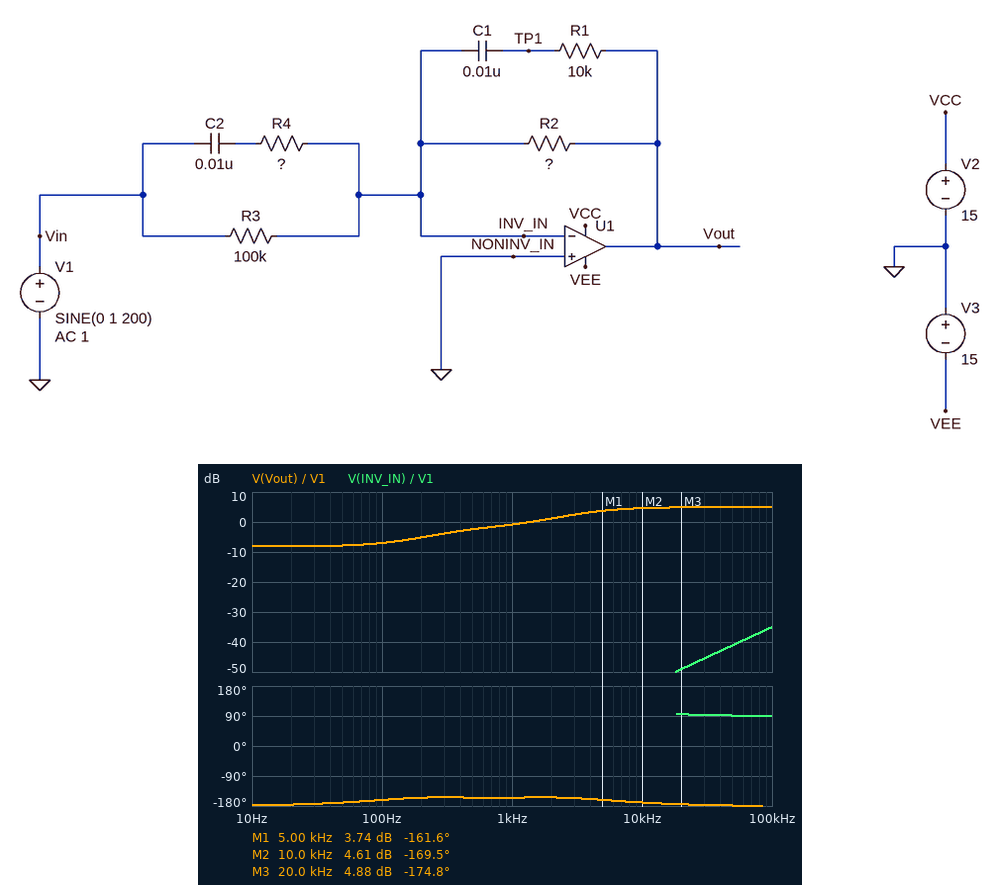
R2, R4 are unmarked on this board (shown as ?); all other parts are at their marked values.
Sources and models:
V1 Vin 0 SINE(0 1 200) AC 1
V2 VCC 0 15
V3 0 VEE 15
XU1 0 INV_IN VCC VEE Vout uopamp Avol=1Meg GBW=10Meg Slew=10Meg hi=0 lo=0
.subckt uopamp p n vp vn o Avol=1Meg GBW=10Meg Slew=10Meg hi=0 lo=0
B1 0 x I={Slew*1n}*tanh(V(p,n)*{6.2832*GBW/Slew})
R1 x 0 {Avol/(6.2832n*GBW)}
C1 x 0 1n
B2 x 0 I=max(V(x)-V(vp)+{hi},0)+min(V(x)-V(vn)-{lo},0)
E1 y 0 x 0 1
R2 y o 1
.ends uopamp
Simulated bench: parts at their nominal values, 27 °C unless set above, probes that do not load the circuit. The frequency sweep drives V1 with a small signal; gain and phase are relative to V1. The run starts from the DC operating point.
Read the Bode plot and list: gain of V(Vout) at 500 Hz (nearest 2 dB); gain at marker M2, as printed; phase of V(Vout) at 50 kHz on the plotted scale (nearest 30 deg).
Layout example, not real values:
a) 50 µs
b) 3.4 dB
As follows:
a) -2 dB
b) 4.61 dB
c) -180 deg
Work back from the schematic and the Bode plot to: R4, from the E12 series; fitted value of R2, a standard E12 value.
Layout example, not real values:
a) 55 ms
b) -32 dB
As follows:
a) 4.7 kΩ
b) 39 kΩ
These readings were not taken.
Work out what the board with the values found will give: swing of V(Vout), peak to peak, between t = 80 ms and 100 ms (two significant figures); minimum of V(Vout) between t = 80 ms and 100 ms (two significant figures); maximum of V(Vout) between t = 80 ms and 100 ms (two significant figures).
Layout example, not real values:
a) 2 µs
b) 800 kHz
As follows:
a) 1.1 V
b) -550 mV
c) 550 mV
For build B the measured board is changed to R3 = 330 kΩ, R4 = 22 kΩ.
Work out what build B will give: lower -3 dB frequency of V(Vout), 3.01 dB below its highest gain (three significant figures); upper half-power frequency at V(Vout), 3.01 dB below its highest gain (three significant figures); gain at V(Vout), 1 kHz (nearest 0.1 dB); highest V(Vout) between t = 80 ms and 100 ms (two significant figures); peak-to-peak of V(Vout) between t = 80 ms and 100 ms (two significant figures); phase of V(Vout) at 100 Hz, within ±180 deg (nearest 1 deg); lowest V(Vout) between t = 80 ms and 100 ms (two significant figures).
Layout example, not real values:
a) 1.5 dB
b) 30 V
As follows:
a) 195 Hz
b) 2.47 kHz
c) -5.0 dB
d) 440 mV
e) 890 mV
f) -136 deg
g) -440 mV
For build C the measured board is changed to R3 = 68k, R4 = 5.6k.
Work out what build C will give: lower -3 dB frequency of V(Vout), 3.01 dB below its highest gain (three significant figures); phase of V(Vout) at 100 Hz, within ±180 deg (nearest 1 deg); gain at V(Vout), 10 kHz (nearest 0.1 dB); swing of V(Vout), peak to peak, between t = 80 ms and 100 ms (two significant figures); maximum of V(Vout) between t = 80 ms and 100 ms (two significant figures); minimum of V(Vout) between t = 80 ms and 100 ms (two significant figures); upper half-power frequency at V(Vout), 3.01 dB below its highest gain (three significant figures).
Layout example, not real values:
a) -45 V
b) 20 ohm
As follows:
a) 1.79 kHz
b) -171 deg
c) 3.5 dB
d) 1.3 V
e) 670 mV
f) -670 mV
g) 3.94 MHz
